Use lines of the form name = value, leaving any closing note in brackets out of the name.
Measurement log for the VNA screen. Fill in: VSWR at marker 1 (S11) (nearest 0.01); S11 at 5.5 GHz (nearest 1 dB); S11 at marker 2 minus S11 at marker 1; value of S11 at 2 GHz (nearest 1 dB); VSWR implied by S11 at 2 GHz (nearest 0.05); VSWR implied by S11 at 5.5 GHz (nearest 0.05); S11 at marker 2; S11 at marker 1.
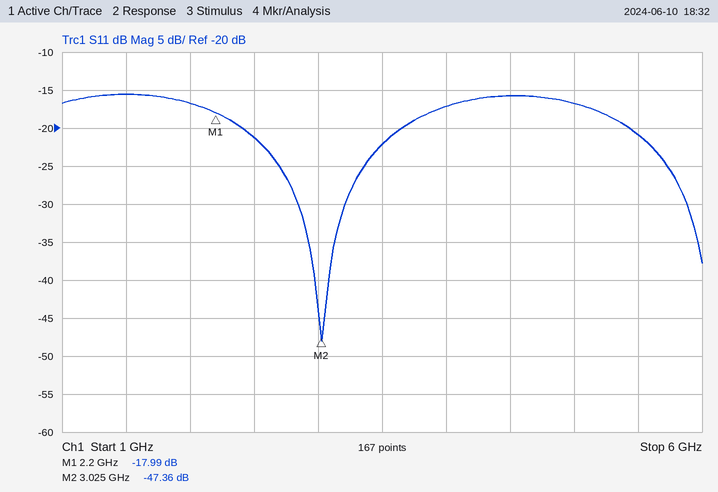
VSWR at marker 1 (S11) = 1.29
S11 at 5.5 GHz = -21 dB
S11 at marker 2 minus S11 at marker 1 = -29.37 dB
value of S11 at 2 GHz = -17 dB
VSWR implied by S11 at 2 GHz = 1.35
VSWR implied by S11 at 5.5 GHz = 1.20
S11 at marker 2 = -47.36 dB
S11 at marker 1 = -17.99 dB
